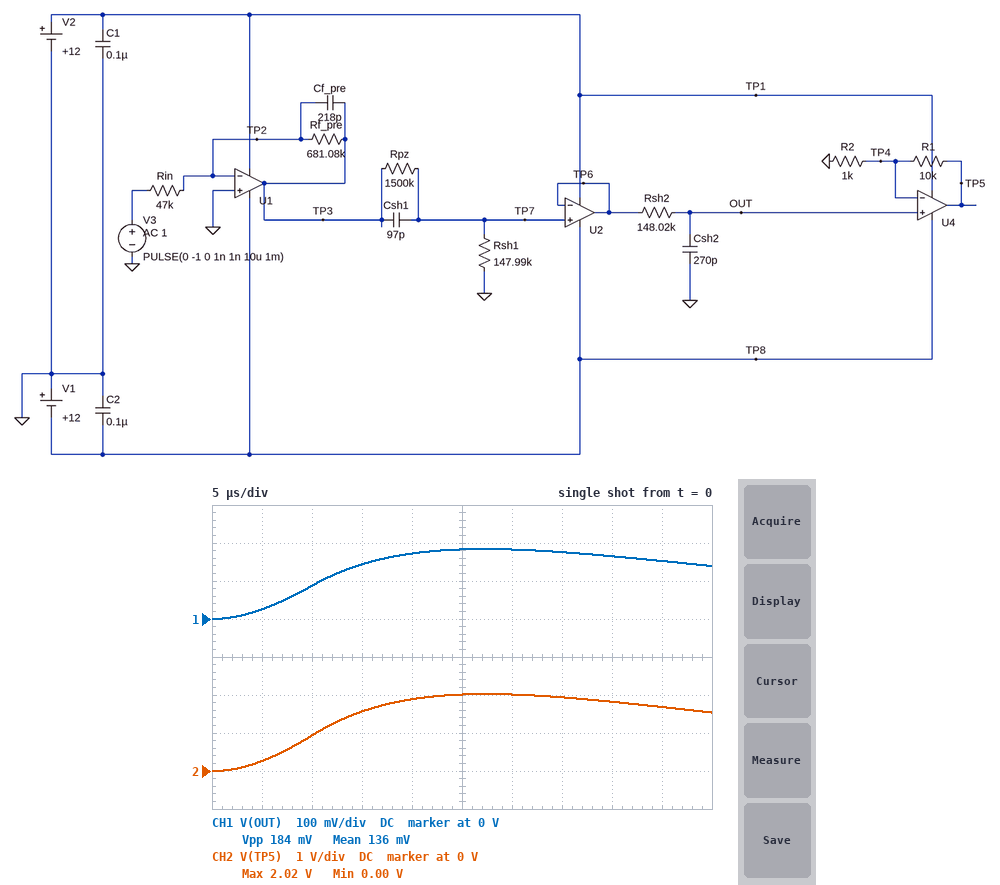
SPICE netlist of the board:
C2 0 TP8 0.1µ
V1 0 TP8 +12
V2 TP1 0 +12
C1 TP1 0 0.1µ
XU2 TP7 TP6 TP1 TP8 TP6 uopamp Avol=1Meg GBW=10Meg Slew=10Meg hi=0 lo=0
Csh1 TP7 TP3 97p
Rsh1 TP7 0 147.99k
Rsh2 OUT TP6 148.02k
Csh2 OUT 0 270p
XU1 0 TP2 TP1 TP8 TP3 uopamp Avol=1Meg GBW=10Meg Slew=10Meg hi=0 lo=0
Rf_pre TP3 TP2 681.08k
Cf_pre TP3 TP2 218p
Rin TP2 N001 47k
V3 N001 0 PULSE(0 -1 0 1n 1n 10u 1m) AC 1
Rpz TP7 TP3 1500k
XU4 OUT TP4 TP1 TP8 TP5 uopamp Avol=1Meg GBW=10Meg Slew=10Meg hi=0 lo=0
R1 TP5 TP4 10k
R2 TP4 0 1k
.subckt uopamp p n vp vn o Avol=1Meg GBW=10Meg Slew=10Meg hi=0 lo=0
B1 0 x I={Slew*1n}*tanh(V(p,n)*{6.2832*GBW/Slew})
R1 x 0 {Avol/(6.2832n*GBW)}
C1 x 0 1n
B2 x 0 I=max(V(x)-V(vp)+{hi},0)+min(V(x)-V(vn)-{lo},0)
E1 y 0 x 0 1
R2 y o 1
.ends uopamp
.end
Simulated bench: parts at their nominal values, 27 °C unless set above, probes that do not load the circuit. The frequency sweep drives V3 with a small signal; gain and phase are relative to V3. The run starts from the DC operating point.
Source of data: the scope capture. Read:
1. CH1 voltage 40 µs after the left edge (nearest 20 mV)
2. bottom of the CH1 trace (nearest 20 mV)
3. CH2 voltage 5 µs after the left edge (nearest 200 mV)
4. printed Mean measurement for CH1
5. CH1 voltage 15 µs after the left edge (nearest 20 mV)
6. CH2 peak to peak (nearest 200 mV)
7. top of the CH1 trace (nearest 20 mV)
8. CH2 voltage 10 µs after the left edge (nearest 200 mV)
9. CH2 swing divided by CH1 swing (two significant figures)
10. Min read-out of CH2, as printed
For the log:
160 mV
0 V
200 mV
136 mV
140 mV
2.0 V
180 mV
1.0 V
11
0.00 V
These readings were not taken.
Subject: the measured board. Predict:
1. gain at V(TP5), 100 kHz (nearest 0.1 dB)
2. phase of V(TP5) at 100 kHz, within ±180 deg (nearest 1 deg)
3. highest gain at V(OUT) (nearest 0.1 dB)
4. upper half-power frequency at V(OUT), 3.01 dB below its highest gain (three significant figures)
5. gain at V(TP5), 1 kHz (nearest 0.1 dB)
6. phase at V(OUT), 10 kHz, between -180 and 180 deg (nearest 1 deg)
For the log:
-23.5 dB
2 deg
2.3 dB
3.51 kHz
22.7 dB
72 deg
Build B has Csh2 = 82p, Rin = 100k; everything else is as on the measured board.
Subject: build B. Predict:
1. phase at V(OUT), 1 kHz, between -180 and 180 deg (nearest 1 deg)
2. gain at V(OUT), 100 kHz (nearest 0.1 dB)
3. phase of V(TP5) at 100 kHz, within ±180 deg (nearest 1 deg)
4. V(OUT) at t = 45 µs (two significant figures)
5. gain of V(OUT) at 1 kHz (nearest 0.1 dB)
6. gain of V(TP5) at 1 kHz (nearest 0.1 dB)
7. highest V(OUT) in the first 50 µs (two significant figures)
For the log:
170 deg
-40.5 dB
7 deg
64 mV
-4.4 dB
16.4 dB
170 mV
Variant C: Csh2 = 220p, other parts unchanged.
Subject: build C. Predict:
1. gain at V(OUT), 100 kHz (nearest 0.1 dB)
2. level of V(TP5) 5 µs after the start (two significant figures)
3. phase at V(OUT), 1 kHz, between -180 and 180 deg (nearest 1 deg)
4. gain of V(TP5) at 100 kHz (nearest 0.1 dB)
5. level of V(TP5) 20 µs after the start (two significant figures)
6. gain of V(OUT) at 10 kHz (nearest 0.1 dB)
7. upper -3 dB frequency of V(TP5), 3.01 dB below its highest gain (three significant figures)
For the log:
-42.5 dB
320 mV
163 deg
-21.7 dB
2.2 V
-7.3 dB
4.15 kHz
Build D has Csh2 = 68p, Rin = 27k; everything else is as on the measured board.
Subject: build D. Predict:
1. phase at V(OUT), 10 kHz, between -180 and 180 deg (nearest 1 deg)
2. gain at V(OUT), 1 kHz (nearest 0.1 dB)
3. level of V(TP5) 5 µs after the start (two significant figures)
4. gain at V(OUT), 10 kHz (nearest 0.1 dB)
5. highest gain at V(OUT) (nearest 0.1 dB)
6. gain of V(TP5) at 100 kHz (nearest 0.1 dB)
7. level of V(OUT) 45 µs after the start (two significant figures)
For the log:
108 deg
7.0 dB
1.6 V
3.2 dB
7.1 dB
-6.8 dB
210 mV
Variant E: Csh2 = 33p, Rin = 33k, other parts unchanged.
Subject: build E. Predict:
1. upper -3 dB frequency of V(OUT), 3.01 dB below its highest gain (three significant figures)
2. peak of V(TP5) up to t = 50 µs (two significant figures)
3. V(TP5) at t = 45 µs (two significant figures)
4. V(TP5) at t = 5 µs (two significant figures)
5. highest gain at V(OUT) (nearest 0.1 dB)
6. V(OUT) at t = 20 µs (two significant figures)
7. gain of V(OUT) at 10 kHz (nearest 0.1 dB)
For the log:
10.4 kHz
8.0 V
1.2 V
2.3 V
5.4 dB
600 mV
2.5 dB
